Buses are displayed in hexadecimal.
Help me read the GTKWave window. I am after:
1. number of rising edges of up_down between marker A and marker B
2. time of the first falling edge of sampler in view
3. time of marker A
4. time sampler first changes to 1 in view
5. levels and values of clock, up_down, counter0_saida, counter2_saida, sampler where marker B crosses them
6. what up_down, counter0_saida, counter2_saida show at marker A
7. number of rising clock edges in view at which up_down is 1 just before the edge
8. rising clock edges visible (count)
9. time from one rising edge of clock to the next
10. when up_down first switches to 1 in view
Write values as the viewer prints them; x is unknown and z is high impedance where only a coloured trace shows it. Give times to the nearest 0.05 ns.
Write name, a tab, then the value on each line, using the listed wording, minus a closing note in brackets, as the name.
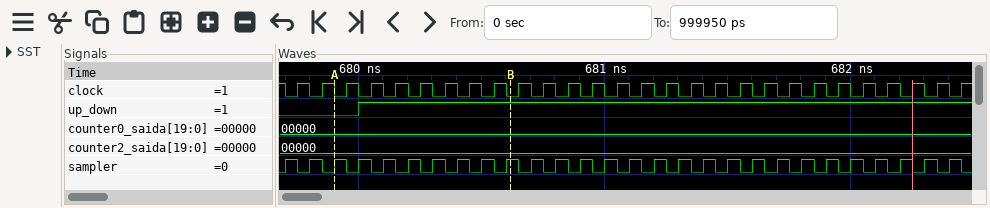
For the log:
number of rising edges of up_down between marker A and marker B	1
time of the first falling edge of sampler in view	679.75 ns
time of marker A	679.9 ns
time sampler first changes to 1 in view	679.7 ns
levels and values of clock, up_down, counter0_saida, counter2_saida, sampler where marker B crosses them	clock=0, up_down=1, counter0_saida=00000, counter2_saida=00000, sampler=1
what up_down, counter0_saida, counter2_saida show at marker A	up_down=0, counter0_saida=00000, counter2_saida=00000
number of rising clock edges in view at which up_down is 1 just before the edge	25
rising clock edges visible	28
time from one rising edge of clock to the next	0.1 ns
when up_down first switches to 1 in view	680 ns
